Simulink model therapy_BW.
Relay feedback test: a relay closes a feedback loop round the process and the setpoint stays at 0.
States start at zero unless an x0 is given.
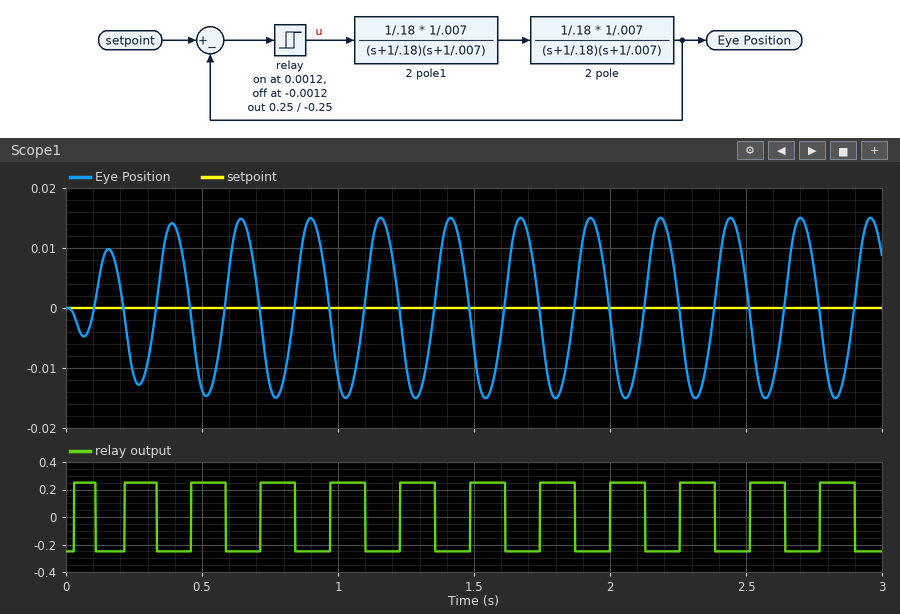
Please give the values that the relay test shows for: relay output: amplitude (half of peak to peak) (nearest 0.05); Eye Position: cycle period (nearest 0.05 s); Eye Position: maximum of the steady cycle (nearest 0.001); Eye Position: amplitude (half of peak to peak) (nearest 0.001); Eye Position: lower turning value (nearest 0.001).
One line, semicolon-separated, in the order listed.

0.25; 0.25 s; 0.015; 0.015; -0.015
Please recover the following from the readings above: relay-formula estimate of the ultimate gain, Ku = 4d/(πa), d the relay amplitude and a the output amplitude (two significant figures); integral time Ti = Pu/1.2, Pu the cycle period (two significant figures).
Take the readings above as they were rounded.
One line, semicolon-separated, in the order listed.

21; 0.21 s
